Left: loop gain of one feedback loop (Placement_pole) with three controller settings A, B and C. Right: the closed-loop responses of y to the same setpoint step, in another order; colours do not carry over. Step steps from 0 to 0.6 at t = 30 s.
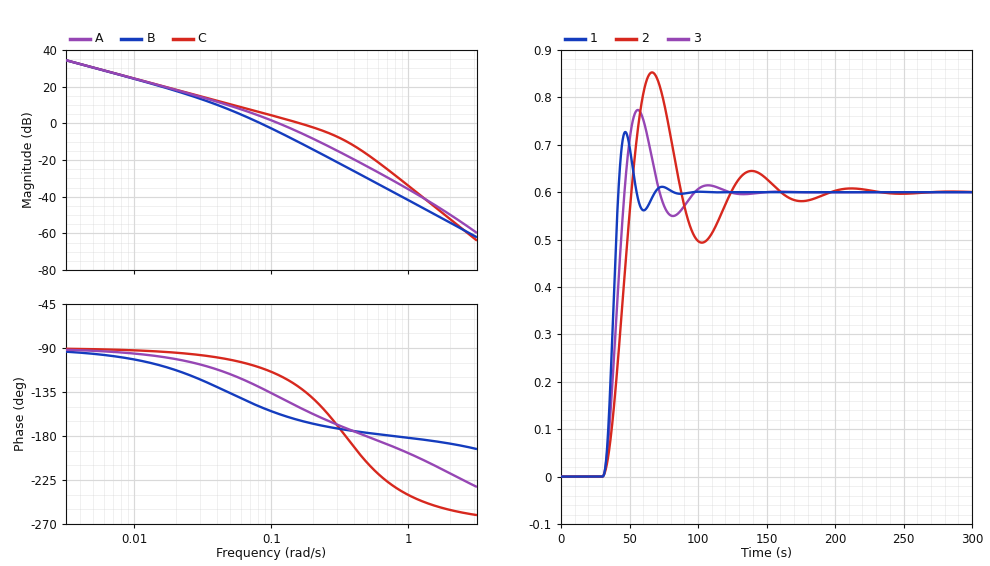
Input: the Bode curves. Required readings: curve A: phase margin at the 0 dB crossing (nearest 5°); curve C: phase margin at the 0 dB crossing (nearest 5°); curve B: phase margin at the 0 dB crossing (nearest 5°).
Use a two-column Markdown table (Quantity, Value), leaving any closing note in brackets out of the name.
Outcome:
| Quantity | Value |
|---|---|
| curve A: phase margin at the 0 dB crossing | 40° |
| curve C: phase margin at the 0 dB crossing | 50° |
| curve B: phase margin at the 0 dB crossing | 30° |
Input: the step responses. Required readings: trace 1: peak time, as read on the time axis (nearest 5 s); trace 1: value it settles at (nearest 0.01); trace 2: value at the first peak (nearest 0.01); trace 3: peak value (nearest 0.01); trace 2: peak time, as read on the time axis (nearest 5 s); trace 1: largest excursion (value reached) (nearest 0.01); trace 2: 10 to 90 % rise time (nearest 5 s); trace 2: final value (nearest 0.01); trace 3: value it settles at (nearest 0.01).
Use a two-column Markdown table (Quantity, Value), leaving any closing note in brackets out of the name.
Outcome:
| Quantity | Value |
|---|---|
| trace 1: peak time, as read on the time axis | 45 s |
| trace 1: value it settles at | 0.60 |
| trace 2: value at the first peak | 0.85 |
| trace 3: peak value | 0.77 |
| trace 2: peak time, as read on the time axis | 65 s |
| trace 1: largest excursion (value reached) | 0.73 |
| trace 2: 10 to 90 % rise time | 15 s |
| trace 2: final value | 0.60 |
| trace 3: value it settles at | 0.60 |
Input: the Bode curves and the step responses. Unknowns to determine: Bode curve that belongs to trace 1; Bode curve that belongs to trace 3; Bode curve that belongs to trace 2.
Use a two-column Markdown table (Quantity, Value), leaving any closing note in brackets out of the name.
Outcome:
| Quantity | Value |
|---|---|
| Bode curve that belongs to trace 1 | C |
| Bode curve that belongs to trace 3 | A |
| Bode curve that belongs to trace 2 | B |
